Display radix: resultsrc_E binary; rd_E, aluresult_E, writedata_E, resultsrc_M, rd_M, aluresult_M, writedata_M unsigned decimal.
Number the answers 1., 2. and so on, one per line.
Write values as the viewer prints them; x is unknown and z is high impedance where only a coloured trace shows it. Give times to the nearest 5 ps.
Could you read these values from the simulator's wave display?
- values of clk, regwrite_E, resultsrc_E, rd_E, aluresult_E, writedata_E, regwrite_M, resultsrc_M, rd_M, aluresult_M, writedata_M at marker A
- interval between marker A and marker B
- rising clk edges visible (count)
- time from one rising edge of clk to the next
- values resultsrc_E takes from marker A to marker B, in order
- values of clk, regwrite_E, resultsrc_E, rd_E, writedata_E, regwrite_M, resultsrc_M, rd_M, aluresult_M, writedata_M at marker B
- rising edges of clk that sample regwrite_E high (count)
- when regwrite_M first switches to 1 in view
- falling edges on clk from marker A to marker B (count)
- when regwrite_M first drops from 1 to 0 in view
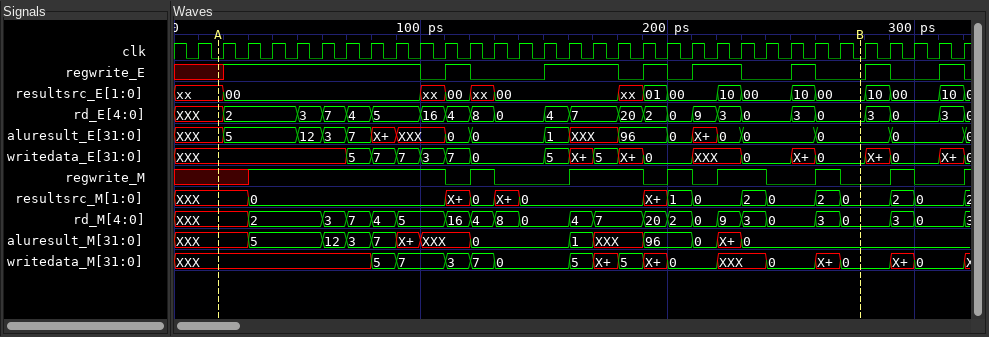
1. clk=0, regwrite_E=x, resultsrc_E=xx, rd_E=XXX, aluresult_E=XXX, writedata_E=XXX, regwrite_M=x, resultsrc_M=XXX, rd_M=XXX, aluresult_M=XXX, writedata_M=XXX
2. 260 ps
3. 32
4. 10 ps
5. xx, 00, xx, 00, xx, 00, xx, 01, 00, 10, 00, 10, 00
6. clk=0, regwrite_E=0, resultsrc_E=00, rd_E=0, writedata_E=0, regwrite_M=0, resultsrc_M=0, rd_M=0, aluresult_M=0, writedata_M=0
7. 18
8. 30 ps
9. 26
10. 110 ps
